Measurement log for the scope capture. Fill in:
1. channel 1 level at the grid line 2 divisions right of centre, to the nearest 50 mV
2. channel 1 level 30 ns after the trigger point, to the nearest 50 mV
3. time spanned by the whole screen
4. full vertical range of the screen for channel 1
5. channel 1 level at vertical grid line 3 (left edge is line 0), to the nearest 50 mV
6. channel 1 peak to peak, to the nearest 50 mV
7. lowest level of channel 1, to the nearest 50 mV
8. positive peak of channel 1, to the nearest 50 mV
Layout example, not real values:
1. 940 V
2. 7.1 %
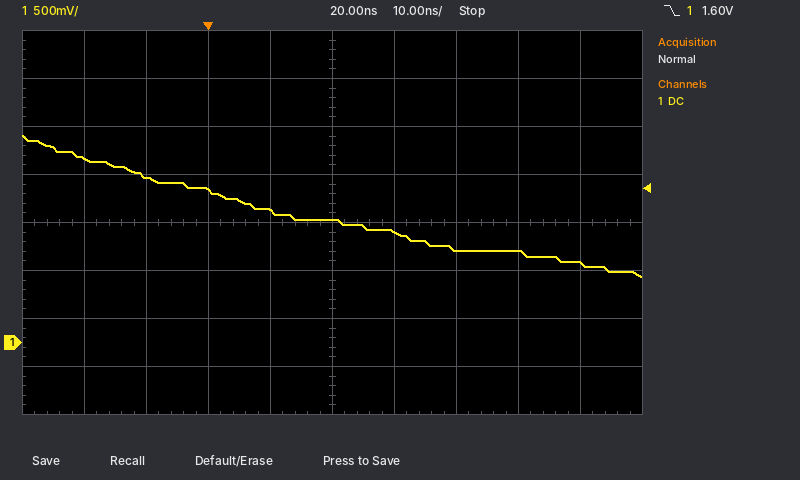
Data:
1. 950 mV
2. 1.15 V
3. 100 ns
4. 4 V
5. 1.60 V
6. 1.45 V
7. 700 mV
8. 2.15 V
